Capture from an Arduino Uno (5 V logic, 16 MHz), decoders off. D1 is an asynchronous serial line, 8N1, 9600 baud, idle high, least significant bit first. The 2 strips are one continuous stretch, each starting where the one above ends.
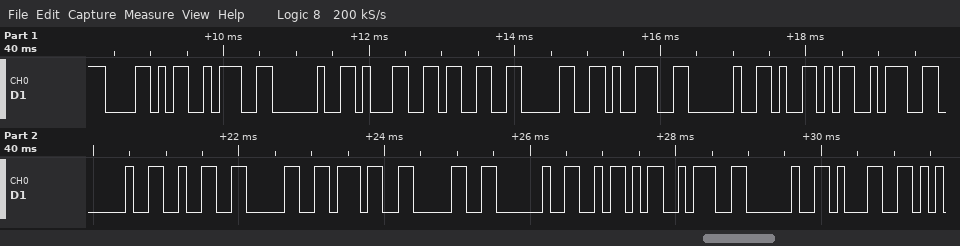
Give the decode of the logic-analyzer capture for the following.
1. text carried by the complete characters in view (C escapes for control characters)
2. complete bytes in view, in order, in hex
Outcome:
"X: 1309 Y: 2070 Z: 1"
58 3A 20 31 33 30 39 20 59 3A 20 32 30 37 30 20 5A 3A 20 31
